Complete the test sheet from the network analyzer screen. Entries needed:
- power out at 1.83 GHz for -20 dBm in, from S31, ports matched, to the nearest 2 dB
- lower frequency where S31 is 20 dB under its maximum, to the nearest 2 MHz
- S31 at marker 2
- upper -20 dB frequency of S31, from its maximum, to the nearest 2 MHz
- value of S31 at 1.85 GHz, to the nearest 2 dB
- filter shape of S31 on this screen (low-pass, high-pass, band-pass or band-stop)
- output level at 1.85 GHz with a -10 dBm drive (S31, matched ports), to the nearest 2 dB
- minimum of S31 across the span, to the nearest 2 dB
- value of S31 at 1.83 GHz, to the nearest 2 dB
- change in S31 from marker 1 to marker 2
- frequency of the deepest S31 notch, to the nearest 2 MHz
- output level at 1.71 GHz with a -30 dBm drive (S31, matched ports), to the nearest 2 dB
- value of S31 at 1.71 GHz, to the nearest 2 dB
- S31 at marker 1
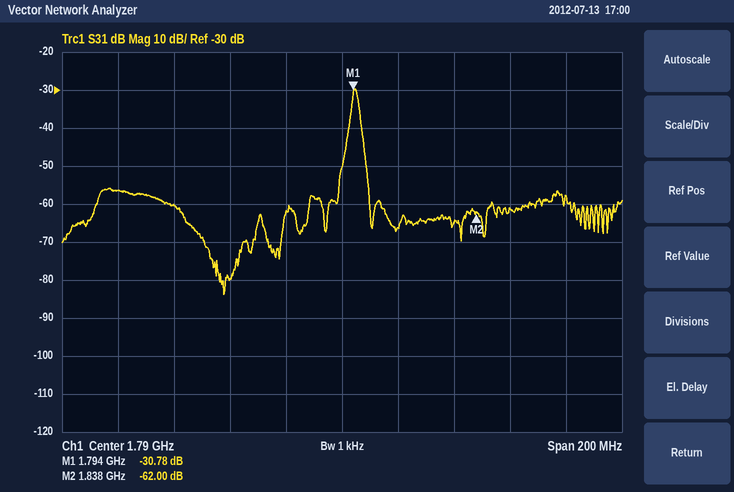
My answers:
-84 dBm
1.790 GHz
-62.00 dB
1.798 GHz
-62 dB
band-pass
-72 dBm
-84 dB
-64 dB
-31.22 dB
1.748 GHz
-86 dBm
-56 dB
-30.78 dB
